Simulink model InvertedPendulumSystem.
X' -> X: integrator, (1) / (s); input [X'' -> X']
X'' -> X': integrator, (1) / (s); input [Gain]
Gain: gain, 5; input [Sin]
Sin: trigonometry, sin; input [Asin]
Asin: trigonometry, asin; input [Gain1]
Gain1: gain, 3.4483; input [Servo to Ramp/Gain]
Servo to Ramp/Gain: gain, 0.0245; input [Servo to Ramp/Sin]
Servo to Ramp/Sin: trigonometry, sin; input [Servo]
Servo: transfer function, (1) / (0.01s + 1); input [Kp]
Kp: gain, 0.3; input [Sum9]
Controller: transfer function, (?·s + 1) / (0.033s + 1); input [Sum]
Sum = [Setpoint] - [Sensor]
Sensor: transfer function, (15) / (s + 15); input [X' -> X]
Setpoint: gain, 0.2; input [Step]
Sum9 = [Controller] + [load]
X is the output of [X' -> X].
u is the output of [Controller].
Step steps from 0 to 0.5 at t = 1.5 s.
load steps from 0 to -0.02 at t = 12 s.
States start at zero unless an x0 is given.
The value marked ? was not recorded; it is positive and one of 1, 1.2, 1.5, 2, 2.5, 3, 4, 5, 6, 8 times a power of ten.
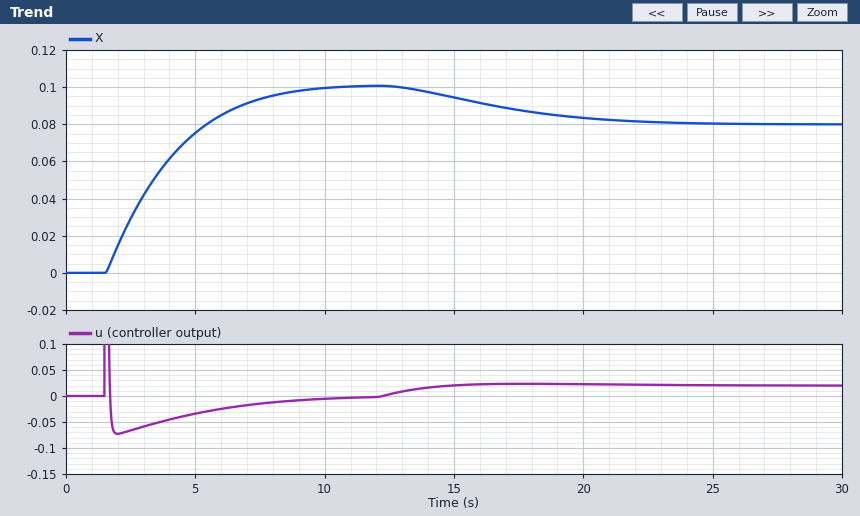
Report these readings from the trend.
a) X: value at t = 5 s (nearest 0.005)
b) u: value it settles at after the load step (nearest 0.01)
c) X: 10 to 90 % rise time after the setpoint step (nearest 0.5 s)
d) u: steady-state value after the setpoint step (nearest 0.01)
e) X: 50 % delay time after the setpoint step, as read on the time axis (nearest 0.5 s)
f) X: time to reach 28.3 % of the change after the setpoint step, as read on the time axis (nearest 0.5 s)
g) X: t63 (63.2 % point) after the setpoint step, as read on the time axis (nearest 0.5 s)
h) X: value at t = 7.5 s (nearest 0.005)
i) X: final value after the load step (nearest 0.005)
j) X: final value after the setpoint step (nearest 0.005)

0.075
0.02
5.0 s
0.00
3.5 s
2.5 s
4.0 s
0.095
0.080
0.100
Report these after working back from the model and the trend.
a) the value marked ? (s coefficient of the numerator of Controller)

5
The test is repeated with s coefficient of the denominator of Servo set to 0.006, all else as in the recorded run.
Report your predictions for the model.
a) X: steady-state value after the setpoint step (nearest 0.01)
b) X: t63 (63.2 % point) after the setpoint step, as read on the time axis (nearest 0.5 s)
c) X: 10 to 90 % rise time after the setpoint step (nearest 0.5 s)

0.10
4.5 s
5.5 s
